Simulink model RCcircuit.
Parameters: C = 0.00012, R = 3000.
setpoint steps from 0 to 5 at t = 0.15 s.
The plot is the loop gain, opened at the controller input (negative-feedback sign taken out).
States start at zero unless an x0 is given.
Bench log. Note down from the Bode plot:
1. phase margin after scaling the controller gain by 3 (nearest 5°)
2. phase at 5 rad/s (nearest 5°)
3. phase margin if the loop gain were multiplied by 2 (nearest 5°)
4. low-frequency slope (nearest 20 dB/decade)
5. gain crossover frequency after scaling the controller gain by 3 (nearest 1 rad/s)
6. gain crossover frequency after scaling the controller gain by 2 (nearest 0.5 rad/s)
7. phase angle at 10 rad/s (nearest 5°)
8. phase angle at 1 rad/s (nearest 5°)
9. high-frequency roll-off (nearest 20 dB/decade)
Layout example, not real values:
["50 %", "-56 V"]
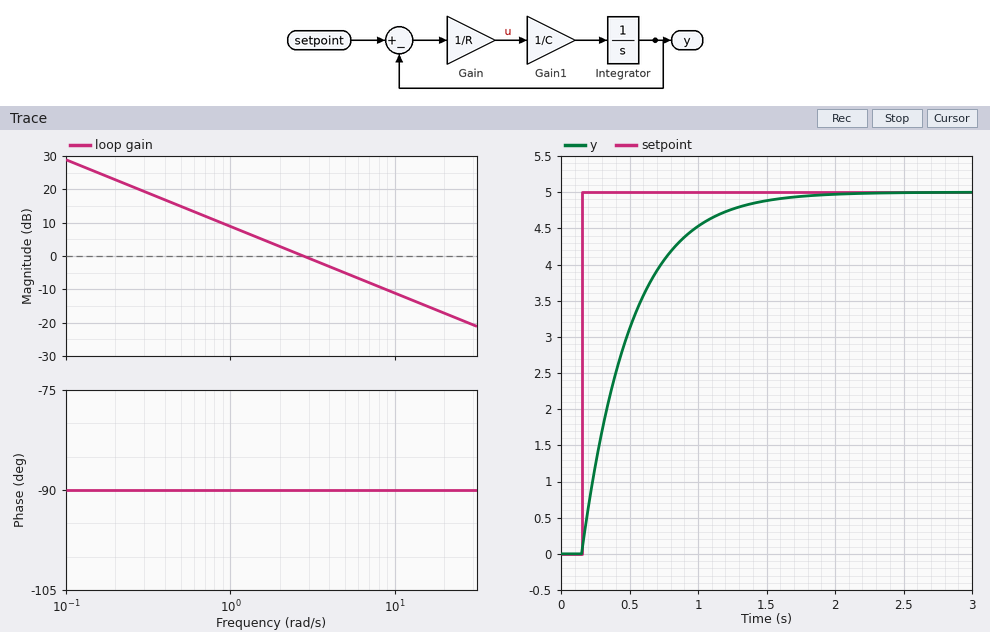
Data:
["90°", "-90°", "90°", "-20 dB/decade", "8 rad/s", "5.5 rad/s", "-90°", "-90°", "-20 dB/decade"]
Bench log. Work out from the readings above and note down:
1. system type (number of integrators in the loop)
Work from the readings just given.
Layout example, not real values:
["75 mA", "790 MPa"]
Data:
["1"]
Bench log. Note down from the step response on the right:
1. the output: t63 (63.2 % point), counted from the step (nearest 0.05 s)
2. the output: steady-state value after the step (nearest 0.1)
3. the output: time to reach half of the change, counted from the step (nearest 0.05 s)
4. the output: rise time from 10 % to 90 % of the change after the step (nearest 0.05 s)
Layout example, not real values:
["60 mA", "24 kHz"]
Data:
["0.35 s", "5.0", "0.25 s", "0.80 s"]
